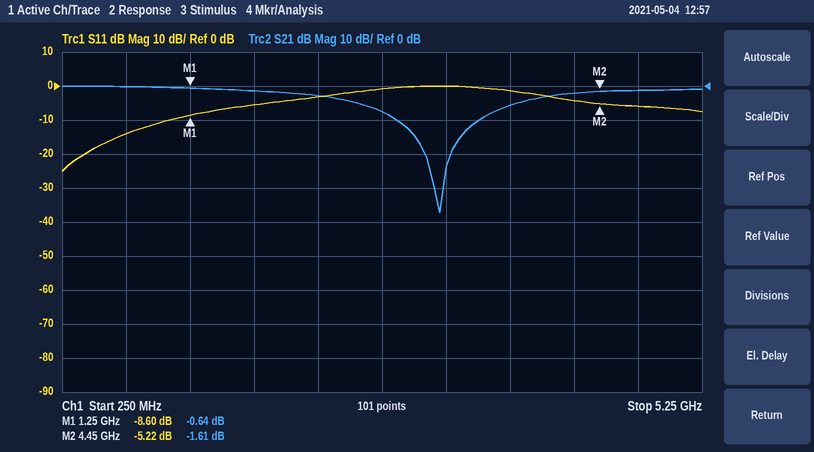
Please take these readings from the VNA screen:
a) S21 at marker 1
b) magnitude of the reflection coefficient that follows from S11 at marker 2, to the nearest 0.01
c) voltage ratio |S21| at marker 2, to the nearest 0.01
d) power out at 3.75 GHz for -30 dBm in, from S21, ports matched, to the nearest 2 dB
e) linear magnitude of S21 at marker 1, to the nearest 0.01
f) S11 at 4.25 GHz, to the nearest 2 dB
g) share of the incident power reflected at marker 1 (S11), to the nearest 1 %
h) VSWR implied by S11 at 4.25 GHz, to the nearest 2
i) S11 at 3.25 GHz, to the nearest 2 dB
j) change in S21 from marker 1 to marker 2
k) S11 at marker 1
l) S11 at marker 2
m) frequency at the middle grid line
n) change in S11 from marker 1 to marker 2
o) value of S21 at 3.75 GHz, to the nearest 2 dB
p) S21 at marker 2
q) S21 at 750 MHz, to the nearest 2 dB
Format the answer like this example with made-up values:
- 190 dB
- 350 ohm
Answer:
- -0.64 dB
- 0.55
- 0.83
- -36 dBm
- 0.93
- -4 dB
- 14 %
- 4
- 0 dB
- -0.97 dB
- -8.60 dB
- -5.22 dB
- 2.75 GHz
- 3.38 dB
- -6 dB
- -1.61 dB
- 0 dB
